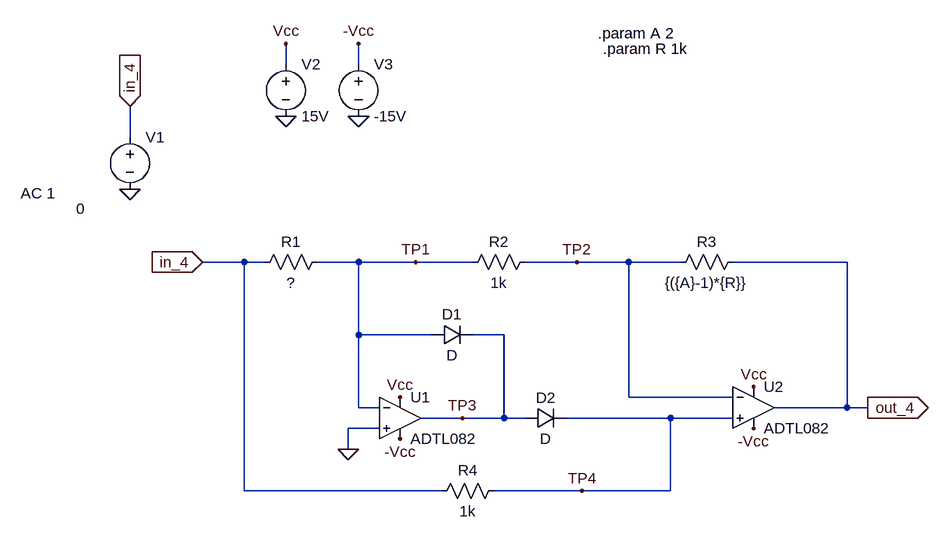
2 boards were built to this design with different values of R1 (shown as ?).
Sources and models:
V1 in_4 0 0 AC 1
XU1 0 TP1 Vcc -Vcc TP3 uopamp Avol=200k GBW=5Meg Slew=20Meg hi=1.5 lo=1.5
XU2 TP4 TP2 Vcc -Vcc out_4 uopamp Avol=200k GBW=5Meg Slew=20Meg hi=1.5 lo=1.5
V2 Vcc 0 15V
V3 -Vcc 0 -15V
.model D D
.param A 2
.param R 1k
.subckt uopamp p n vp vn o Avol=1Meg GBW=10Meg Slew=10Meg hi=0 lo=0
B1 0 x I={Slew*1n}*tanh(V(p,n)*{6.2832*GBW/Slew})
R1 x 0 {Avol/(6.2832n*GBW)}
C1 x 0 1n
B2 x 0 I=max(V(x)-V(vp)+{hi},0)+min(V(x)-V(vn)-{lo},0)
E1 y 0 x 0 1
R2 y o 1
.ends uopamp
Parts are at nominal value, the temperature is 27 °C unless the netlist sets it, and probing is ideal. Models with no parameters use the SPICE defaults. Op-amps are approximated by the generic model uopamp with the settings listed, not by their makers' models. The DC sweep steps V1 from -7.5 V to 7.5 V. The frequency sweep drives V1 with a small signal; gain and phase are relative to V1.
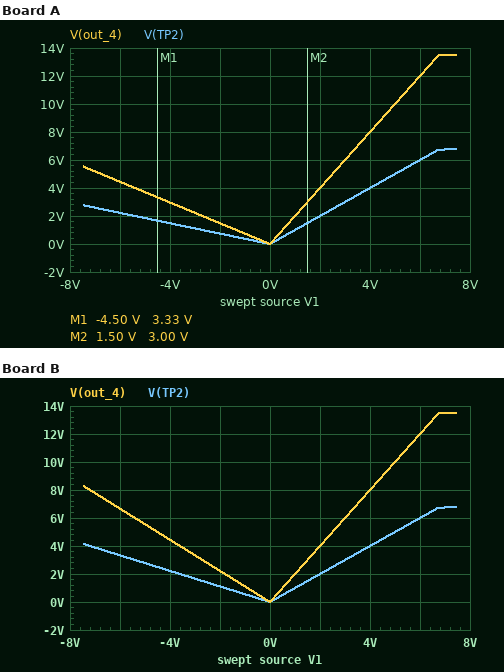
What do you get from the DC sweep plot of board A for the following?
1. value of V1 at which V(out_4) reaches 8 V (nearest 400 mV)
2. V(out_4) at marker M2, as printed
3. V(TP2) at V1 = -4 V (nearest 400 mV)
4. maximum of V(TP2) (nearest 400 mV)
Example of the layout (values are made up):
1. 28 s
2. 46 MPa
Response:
1. 4.0 V
2. 3.00 V
3. 1.6 V
4. 6.8 V
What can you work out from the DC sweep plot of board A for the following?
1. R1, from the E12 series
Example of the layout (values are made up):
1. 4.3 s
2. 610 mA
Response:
1. 2.7 kΩ
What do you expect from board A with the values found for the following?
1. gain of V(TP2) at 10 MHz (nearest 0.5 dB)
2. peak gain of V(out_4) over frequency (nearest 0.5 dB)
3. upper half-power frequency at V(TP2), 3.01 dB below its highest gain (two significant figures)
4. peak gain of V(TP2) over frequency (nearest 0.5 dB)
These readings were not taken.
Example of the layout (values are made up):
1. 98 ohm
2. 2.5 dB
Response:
1. -7.5 dB
2. 0 dB
3. 4.1 MHz
4. 0 dB
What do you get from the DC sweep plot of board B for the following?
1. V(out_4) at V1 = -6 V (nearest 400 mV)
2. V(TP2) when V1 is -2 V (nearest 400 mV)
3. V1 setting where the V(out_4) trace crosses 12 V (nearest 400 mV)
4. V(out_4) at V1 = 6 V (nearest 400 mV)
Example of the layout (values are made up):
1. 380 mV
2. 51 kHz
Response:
1. 6.8 V
2. 1.2 V
3. 6.0 V
4. 12.0 V
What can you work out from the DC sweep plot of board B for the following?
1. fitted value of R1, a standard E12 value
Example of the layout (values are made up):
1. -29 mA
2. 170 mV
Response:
1. 1.8 kΩ
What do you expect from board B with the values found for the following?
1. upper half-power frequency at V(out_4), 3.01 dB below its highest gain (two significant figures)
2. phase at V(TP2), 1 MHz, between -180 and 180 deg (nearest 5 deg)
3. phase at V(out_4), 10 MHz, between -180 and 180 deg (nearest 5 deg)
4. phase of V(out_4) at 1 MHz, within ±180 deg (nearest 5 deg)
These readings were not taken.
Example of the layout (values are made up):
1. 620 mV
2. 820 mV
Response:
1. 3.7 MHz
2. -10 deg
3. -70 deg
4. -15 deg
